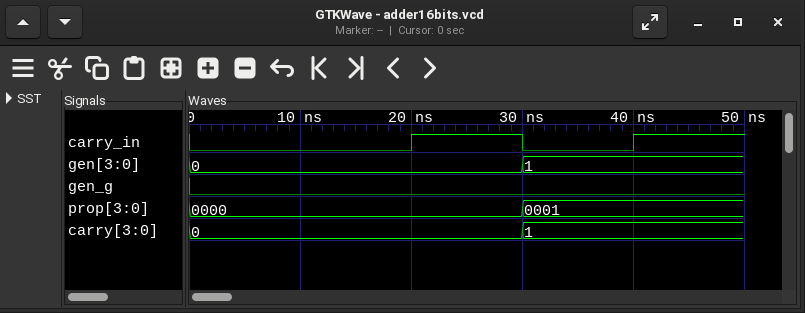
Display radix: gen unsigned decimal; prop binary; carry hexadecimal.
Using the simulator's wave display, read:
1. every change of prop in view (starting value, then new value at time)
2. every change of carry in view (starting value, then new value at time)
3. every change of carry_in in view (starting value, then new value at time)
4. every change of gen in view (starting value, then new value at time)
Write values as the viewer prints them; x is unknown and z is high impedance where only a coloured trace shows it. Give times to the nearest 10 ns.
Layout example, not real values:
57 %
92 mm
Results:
0000, 0001 at 30 ns
0, 1 at 30 ns
0, 1 at 20 ns, 0 at 30 ns, 1 at 40 ns
0, 1 at 30 ns
